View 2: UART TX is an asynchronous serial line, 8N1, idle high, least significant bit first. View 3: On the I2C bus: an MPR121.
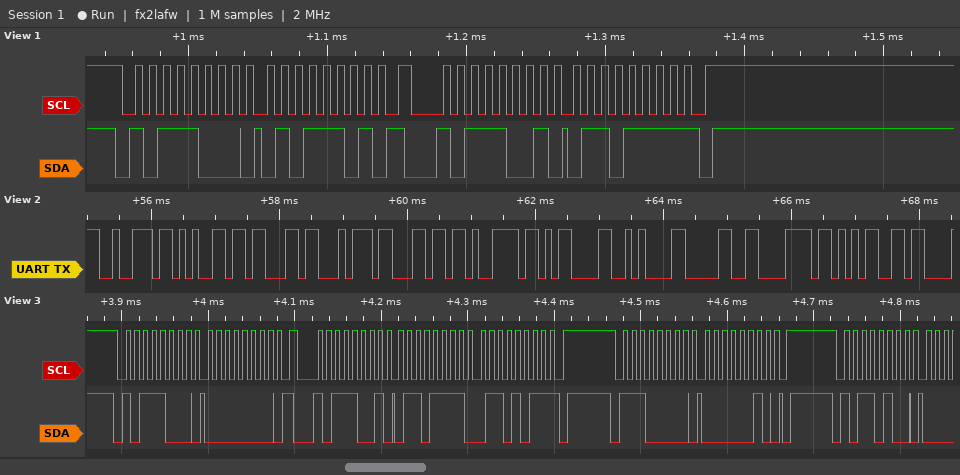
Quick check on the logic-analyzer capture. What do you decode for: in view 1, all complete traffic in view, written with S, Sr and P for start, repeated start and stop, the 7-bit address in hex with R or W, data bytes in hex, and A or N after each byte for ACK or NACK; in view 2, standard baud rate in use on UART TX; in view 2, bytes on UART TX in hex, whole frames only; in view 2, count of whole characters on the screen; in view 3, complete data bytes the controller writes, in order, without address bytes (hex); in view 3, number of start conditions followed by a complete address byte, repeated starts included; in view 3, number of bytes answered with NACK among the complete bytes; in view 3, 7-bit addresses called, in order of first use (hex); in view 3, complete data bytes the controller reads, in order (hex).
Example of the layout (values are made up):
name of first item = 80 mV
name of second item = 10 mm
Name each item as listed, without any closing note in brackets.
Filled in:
in view 1, all complete traffic in view, written with S, Sr and P for start, repeated start and stop, the 7-bit address in hex with R or W, data bytes in hex, and A or N after each byte for ACK or NACK = S 5CW A 5D A Sr 5CR A 6F N P
in view 2, standard baud rate in use on UART TX = 9600 baud
in view 2, bytes on UART TX in hex, whole frames only = 0x72 0x65 0x63 0x74 0x6C 0x79 0x0D 0x0A 0x30 0x78 0x35
in view 2, count of whole characters on the screen = 11
in view 3, complete data bytes the controller writes, in order, without address bytes = 00 02
in view 3, number of start conditions followed by a complete address byte, repeated starts included = 4
in view 3, number of bytes answered with NACK among the complete bytes = 1
in view 3, 7-bit addresses called, in order of first use = 0x5C 0x70 0x5A
in view 3, complete data bytes the controller reads, in order = 6F 6B
